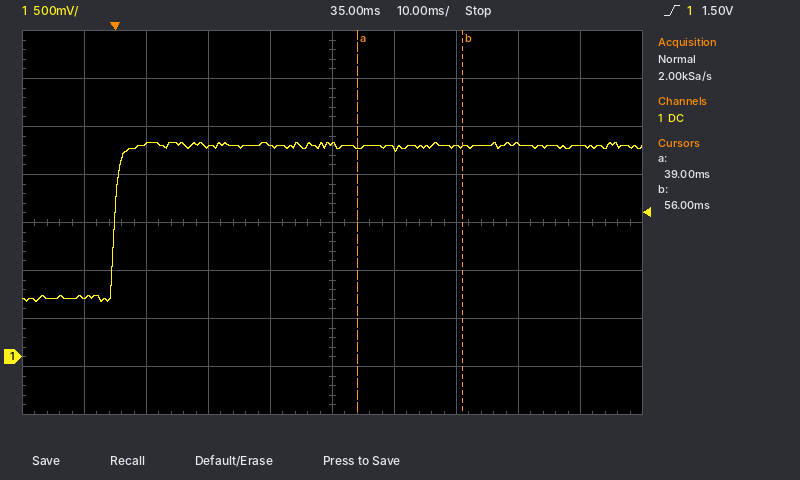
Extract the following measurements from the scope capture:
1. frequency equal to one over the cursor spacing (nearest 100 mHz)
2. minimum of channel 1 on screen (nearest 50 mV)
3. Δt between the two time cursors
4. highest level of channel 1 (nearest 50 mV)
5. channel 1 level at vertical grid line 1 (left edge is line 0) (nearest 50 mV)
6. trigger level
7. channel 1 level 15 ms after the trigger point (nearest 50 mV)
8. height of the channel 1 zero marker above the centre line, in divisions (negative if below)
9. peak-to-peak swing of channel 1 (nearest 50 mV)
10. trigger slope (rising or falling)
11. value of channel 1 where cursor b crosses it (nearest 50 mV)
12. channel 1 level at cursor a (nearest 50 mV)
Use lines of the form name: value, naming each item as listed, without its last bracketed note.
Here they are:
frequency equal to one over the cursor spacing: 58.8 Hz
minimum of channel 1 on screen: 600 mV
Δt between the two time cursors: 17 ms
highest level of channel 1: 2.25 V
channel 1 level at vertical grid line 1 (left edge is line 0): 600 mV
trigger level: 1.50 V
channel 1 level 15 ms after the trigger point: 2.20 V
height of the channel 1 zero marker above the centre line, in divisions: -2.8 div
peak-to-peak swing of channel 1: 1.65 V
trigger slope: rising
value of channel 1 where cursor b crosses it: 2.20 V
channel 1 level at cursor a: 2.20 V
